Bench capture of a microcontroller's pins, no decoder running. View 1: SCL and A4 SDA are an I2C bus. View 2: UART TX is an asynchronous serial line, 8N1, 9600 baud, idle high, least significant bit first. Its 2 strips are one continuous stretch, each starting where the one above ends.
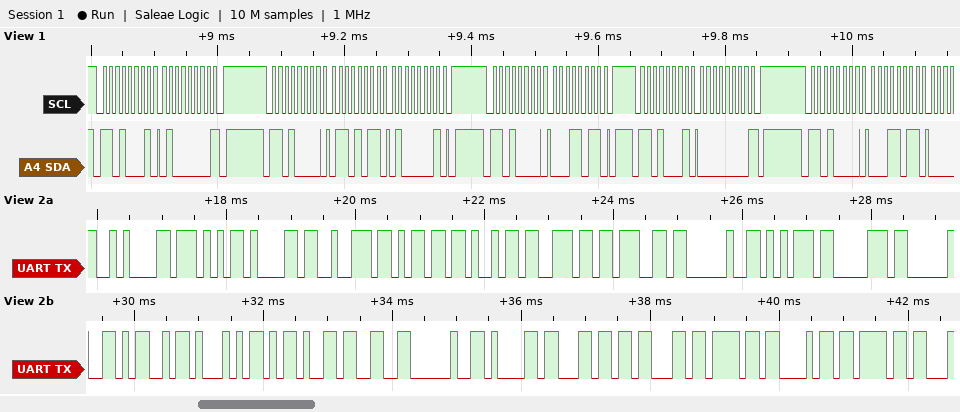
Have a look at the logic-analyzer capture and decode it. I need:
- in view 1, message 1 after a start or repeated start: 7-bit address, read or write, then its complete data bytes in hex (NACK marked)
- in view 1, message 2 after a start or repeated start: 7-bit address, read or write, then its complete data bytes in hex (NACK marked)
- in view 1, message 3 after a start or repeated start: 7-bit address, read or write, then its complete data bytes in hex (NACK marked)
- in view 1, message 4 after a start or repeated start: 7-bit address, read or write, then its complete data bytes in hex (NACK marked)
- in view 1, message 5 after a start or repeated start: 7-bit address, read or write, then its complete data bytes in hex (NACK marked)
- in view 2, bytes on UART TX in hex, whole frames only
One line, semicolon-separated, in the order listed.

0x68 read: 40 NACK; 0x68 write: 6B 41; 0x68 write: 1B; 0x68 read: 00 NACK; 0x68 write: 1B; 0A 57 61 72 6D 69 6E 67 20 75 70 20 4D 51 2D 33 20 61 6C 63 6F 68 6F
